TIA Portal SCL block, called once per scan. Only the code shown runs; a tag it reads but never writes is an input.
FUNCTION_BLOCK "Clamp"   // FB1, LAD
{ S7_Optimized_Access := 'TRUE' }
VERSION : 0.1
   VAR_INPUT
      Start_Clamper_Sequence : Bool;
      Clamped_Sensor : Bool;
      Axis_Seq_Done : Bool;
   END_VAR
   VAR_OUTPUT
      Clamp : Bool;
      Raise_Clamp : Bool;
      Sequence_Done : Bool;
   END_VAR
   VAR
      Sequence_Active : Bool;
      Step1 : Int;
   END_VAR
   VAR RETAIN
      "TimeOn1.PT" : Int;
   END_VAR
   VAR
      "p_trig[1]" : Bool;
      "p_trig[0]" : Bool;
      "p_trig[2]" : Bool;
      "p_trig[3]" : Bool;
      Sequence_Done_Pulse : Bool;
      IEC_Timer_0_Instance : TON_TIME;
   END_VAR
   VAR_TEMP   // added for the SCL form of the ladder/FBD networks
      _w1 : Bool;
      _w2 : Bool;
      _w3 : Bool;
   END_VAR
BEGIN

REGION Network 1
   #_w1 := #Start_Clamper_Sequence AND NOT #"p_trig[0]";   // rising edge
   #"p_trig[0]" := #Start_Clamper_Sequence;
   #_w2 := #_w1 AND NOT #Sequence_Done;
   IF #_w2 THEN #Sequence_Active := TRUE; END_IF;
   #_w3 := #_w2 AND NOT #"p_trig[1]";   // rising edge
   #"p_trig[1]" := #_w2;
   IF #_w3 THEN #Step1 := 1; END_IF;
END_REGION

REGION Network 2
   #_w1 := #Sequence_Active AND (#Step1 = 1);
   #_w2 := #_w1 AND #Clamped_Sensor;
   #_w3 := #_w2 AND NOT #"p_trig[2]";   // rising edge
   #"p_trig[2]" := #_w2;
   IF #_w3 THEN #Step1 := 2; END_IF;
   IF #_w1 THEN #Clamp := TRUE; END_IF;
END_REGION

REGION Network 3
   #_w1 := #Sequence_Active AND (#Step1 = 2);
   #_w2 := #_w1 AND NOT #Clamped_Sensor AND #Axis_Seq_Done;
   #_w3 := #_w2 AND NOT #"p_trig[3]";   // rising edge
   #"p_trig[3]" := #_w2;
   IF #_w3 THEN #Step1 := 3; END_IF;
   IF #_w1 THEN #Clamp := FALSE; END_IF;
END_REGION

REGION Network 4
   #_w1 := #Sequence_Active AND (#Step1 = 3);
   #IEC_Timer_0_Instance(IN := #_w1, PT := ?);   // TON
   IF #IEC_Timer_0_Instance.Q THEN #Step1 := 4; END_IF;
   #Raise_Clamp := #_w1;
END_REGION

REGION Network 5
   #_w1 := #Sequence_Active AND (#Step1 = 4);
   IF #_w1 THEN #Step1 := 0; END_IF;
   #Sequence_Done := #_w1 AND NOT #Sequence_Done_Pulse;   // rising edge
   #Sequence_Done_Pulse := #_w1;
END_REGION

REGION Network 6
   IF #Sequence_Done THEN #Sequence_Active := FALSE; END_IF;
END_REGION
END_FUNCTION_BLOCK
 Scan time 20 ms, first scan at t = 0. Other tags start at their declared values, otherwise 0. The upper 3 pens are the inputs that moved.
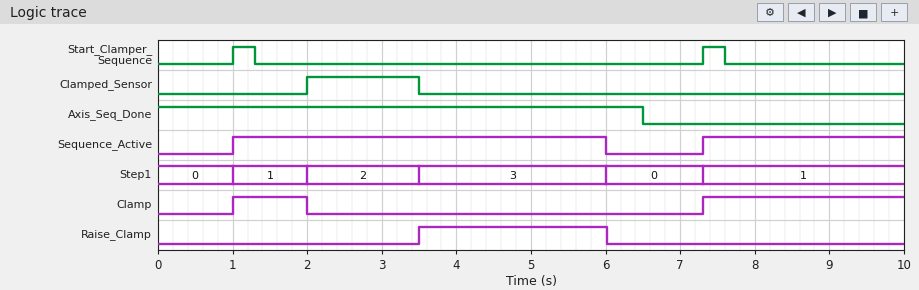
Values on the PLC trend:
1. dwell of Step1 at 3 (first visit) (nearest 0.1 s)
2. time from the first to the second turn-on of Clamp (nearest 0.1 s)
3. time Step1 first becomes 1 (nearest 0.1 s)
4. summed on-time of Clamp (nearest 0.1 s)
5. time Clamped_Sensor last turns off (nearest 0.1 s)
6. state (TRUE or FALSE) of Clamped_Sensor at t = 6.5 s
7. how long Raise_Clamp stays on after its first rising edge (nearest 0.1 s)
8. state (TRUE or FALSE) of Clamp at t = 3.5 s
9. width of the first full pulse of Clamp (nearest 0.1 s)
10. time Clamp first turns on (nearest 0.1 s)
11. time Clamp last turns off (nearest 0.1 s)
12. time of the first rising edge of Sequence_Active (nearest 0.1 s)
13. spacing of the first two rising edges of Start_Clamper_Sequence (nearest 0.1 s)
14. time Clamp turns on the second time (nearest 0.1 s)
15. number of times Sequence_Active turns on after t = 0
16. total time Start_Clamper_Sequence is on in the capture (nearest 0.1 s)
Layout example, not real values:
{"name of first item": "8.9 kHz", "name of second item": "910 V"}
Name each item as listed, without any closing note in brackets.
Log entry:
{"dwell of Step1 at 3 (first visit)": "2.5 s", "time from the first to the second turn-on of Clamp": "6.3 s", "time Step1 first becomes 1": "1.0 s", "summed on-time of Clamp": "3.7 s", "time Clamped_Sensor last turns off": "3.5 s", "state (TRUE or FALSE) of Clamped_Sensor at t = 6.5 s": "FALSE", "how long Raise_Clamp stays on after its first rising edge": "2.5 s", "state (TRUE or FALSE) of Clamp at t = 3.5 s": "FALSE", "width of the first full pulse of Clamp": "1.0 s", "time Clamp first turns on": "1.0 s", "time Clamp last turns off": "2.0 s", "time of the first rising edge of Sequence_Active": "1.0 s", "spacing of the first two rising edges of Start_Clamper_Sequence": "6.3 s", "time Clamp turns on the second time": "7.3 s", "number of times Sequence_Active turns on after t = 0": "2", "total time Start_Clamper_Sequence is on in the capture": "0.6 s"}
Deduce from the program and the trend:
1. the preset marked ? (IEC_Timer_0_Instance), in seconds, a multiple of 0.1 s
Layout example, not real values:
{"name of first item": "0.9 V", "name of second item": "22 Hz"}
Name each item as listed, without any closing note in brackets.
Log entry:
{"the preset marked ? (IEC_Timer_0_Instance), in seconds, a multiple of 0.1 s": "2.5 s"}
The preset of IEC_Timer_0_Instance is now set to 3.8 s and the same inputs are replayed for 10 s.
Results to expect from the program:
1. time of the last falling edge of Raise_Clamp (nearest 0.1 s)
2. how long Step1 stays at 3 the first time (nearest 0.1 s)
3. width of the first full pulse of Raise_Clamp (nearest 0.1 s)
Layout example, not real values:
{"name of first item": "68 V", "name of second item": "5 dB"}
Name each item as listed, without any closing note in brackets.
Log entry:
{"time of the last falling edge of Raise_Clamp": "7.3 s", "how long Step1 stays at 3 the first time": "3.8 s", "width of the first full pulse of Raise_Clamp": "3.8 s"}
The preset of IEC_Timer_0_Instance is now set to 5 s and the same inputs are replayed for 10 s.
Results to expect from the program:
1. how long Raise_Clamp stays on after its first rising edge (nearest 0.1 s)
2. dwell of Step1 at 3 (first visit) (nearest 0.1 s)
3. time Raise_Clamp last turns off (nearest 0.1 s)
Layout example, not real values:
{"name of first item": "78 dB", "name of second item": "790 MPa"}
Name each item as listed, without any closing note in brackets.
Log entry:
{"how long Raise_Clamp stays on after its first rising edge": "3.8 s", "dwell of Step1 at 3 (first visit)": "3.8 s", "time Raise_Clamp last turns off": "7.3 s"}
